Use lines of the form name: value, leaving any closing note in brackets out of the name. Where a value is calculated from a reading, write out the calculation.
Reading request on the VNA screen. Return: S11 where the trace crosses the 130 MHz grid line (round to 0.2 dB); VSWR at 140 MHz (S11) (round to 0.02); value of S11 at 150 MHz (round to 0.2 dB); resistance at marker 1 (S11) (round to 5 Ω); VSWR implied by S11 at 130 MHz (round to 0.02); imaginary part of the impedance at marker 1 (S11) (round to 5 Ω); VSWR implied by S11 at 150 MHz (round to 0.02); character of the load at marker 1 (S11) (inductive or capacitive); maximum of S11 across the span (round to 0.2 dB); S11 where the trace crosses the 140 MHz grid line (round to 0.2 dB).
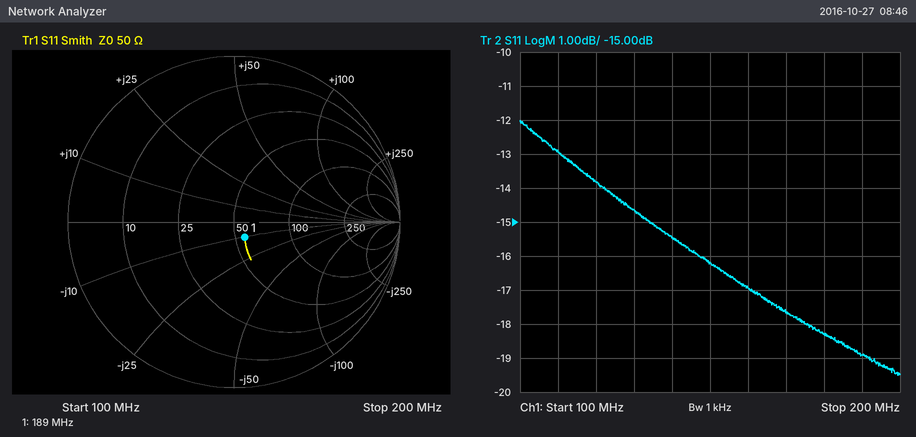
S11 where the trace crosses the 130 MHz grid line: -14.6 dB
VSWR at 140 MHz (S11): |Γ| = 10^(-15.4/20) = 0.1698; VSWR = (1 + 0.1698)/(1 − 0.1698) ≈ 1.41, so 1.40 to the nearest 0.02
value of S11 at 150 MHz: -16.2 dB
resistance at marker 1 (S11): 55 Ω
VSWR implied by S11 at 130 MHz: |Γ| = 10^(-14.6/20) = 0.1862; VSWR = (1 + 0.1862)/(1 − 0.1862) ≈ 1.46
imaginary part of the impedance at marker 1 (S11): -10 Ω
VSWR implied by S11 at 150 MHz: |Γ| = 10^(-16.2/20) = 0.1549; VSWR = (1 + 0.1549)/(1 − 0.1549) ≈ 1.37, so 1.36 to the nearest 0.02
character of the load at marker 1 (S11): capacitive
maximum of S11 across the span: -12.0 dB
S11 where the trace crosses the 140 MHz grid line: -15.4 dB
